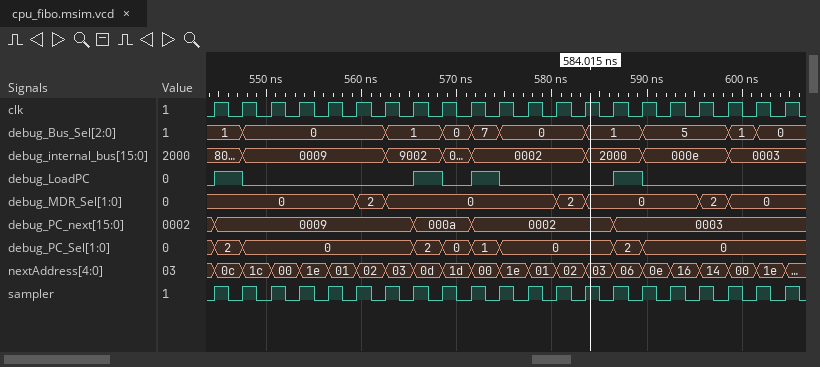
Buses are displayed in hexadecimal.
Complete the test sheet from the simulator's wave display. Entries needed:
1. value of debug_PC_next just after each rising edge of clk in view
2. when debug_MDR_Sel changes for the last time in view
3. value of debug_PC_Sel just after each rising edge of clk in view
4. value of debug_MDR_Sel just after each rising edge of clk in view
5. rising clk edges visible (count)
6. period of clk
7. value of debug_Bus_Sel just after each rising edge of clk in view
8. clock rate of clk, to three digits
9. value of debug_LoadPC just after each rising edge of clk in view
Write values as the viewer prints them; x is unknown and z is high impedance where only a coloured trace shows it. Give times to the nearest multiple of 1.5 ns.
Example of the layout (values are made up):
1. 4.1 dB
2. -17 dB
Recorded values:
1. 0009, 0009, 0009, 0009, 0009, 0009, 0009, 000a, 000a, 0002, 0002, 0002, 0002, 0002, 0003, 0003, 0003, 0003, 0003, 0003, 0003
2. 598.5 ns
3. 2, 0, 0, 0, 0, 0, 0, 2, 0, 1, 0, 0, 0, 0, 2, 0, 0, 0, 0, 0, 0
4. 0, 0, 0, 0, 0, 2, 0, 0, 0, 0, 0, 0, 2, 0, 0, 0, 0, 2, 0, 0, 0
5. 21
6. 3 ns
7. 1, 0, 0, 0, 0, 0, 1, 1, 0, 7, 0, 0, 0, 1, 1, 5, 5, 5, 1, 0, 0
8. 333 MHz
9. 1 0 0 0 0 0 0 1 0 1 0 0 0 0 1 0 0 0 0 0 0
